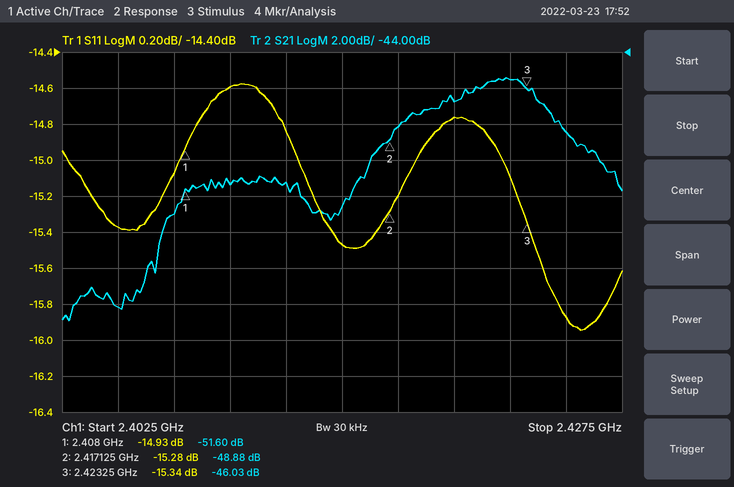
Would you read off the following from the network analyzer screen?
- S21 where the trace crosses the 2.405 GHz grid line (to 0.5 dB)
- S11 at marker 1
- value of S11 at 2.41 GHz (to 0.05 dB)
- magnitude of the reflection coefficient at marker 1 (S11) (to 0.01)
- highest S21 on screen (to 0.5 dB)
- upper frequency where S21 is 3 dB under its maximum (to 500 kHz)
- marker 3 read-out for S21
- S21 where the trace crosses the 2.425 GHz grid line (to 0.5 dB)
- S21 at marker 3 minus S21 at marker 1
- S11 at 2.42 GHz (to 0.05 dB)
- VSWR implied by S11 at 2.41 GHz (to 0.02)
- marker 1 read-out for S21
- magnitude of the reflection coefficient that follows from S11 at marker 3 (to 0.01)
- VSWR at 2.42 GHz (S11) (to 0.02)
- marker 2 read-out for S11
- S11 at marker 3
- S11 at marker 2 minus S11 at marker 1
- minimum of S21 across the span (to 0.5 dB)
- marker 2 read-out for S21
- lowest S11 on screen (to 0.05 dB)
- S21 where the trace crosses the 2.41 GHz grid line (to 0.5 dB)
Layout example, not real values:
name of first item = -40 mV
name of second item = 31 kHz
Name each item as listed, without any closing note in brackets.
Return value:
S21 where the trace crosses the 2.405 GHz grid line = -58.0 dB
S11 at marker 1 = -14.93 dB
value of S11 at 2.41 GHz = -14.60 dB
magnitude of the reflection coefficient at marker 1 (S11) = 0.18
highest S21 on screen = -45.5 dB
upper frequency where S21 is 3 dB under its maximum = 2.4250 GHz
marker 3 read-out for S21 = -46.03 dB
S21 where the trace crosses the 2.425 GHz grid line = -48.5 dB
S21 at marker 3 minus S21 at marker 1 = 5.57 dB
S11 at 2.42 GHz = -14.75 dB
VSWR implied by S11 at 2.41 GHz = 1.46
marker 1 read-out for S21 = -51.60 dB
magnitude of the reflection coefficient that follows from S11 at marker 3 = 0.17
VSWR at 2.42 GHz (S11) = 1.44
marker 2 read-out for S11 = -15.28 dB
S11 at marker 3 = -15.34 dB
S11 at marker 2 minus S11 at marker 1 = -0.35 dB
minimum of S21 across the span = -59.0 dB
marker 2 read-out for S21 = -48.88 dB
lowest S11 on screen = -15.95 dB
S21 where the trace crosses the 2.41 GHz grid line = -51.5 dB
